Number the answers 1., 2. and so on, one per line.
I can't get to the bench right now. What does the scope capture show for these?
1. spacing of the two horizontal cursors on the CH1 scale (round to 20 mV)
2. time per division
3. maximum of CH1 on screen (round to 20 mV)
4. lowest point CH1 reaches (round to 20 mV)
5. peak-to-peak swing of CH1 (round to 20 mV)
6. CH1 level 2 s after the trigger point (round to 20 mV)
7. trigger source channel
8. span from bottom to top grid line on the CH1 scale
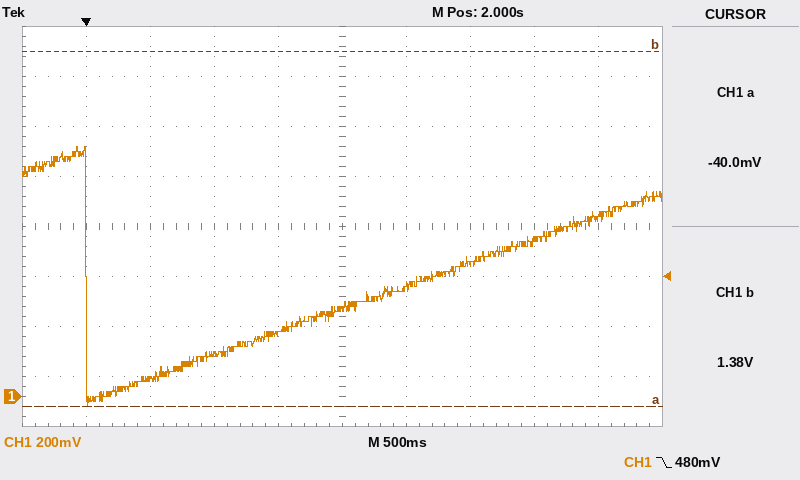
1. 1.42 V
2. 500 ms
3. 1.00 V
4. -40 mV
5. 1.04 V
6. 360 mV
7. CH1
8. 1.6 V
